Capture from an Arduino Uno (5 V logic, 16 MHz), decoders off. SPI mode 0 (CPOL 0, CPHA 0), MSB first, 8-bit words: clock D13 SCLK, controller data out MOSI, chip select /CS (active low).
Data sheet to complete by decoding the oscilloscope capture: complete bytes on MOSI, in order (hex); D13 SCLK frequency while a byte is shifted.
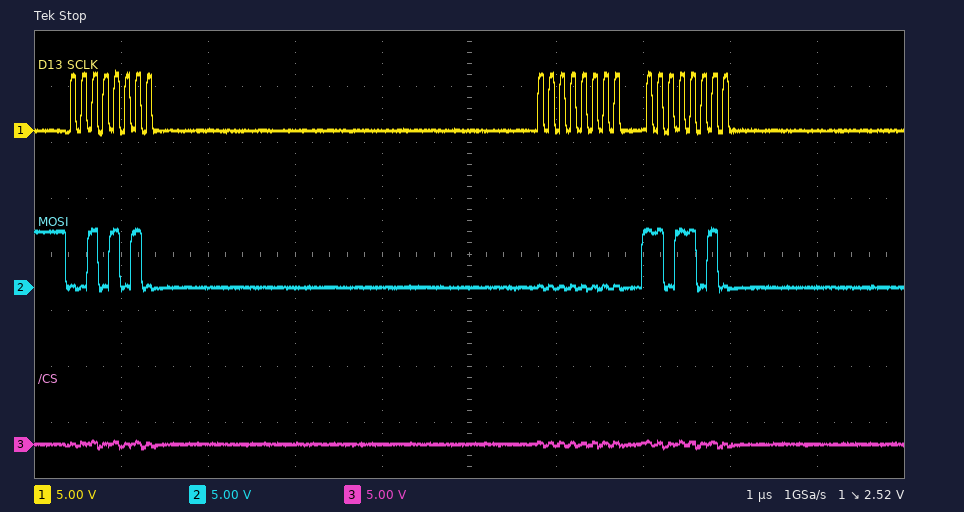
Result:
2A 00 DA
8 MHz
